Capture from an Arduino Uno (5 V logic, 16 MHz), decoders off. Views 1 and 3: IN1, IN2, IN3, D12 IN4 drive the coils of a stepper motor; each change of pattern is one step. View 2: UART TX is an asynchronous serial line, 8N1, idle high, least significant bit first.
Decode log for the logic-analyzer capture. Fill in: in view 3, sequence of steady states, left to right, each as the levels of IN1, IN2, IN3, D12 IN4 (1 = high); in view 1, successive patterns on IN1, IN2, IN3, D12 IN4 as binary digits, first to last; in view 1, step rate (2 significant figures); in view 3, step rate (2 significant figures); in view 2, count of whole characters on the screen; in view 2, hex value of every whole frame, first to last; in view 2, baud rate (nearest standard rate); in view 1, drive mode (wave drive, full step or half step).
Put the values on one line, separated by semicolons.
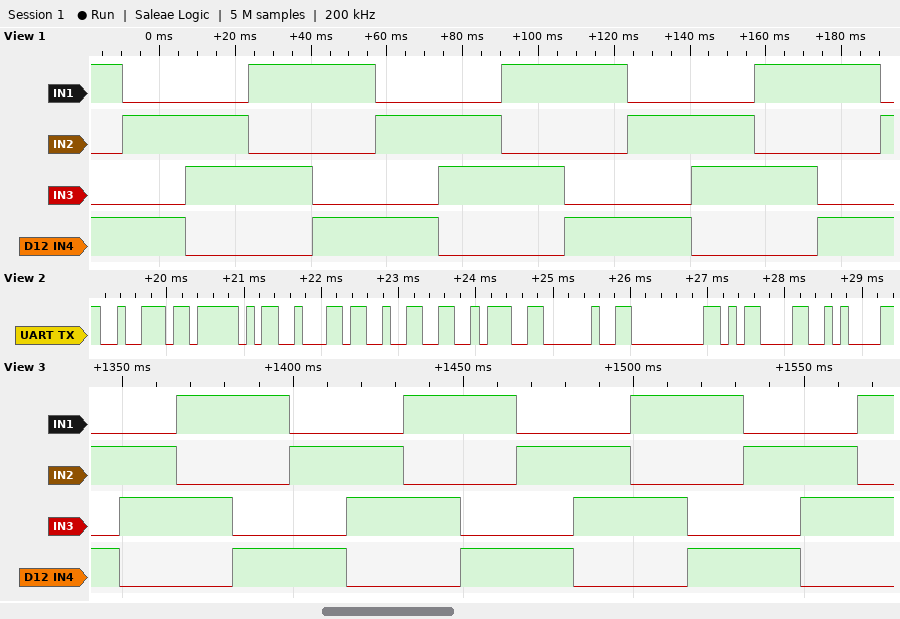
0101 0110 1010 1001 0101 0110 1010 1001 0101 0110 1010 1001 0101 0110 1010; 1001 0101 0110 1010 1001 0101 0110 1010 1001 0101 0110 1010 1001 0101; 60 steps/s; 60 steps/s; 9; 0x72 0x5F 0x62 0x32 0x3A 0x20 0x00 0x0D 0x0A; 9600 baud; full step
